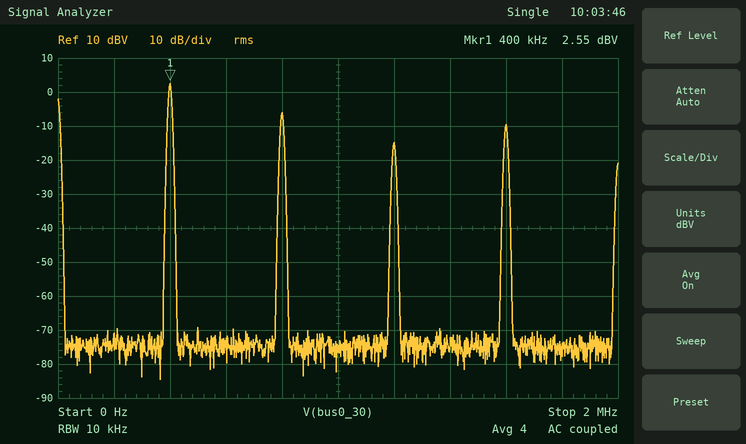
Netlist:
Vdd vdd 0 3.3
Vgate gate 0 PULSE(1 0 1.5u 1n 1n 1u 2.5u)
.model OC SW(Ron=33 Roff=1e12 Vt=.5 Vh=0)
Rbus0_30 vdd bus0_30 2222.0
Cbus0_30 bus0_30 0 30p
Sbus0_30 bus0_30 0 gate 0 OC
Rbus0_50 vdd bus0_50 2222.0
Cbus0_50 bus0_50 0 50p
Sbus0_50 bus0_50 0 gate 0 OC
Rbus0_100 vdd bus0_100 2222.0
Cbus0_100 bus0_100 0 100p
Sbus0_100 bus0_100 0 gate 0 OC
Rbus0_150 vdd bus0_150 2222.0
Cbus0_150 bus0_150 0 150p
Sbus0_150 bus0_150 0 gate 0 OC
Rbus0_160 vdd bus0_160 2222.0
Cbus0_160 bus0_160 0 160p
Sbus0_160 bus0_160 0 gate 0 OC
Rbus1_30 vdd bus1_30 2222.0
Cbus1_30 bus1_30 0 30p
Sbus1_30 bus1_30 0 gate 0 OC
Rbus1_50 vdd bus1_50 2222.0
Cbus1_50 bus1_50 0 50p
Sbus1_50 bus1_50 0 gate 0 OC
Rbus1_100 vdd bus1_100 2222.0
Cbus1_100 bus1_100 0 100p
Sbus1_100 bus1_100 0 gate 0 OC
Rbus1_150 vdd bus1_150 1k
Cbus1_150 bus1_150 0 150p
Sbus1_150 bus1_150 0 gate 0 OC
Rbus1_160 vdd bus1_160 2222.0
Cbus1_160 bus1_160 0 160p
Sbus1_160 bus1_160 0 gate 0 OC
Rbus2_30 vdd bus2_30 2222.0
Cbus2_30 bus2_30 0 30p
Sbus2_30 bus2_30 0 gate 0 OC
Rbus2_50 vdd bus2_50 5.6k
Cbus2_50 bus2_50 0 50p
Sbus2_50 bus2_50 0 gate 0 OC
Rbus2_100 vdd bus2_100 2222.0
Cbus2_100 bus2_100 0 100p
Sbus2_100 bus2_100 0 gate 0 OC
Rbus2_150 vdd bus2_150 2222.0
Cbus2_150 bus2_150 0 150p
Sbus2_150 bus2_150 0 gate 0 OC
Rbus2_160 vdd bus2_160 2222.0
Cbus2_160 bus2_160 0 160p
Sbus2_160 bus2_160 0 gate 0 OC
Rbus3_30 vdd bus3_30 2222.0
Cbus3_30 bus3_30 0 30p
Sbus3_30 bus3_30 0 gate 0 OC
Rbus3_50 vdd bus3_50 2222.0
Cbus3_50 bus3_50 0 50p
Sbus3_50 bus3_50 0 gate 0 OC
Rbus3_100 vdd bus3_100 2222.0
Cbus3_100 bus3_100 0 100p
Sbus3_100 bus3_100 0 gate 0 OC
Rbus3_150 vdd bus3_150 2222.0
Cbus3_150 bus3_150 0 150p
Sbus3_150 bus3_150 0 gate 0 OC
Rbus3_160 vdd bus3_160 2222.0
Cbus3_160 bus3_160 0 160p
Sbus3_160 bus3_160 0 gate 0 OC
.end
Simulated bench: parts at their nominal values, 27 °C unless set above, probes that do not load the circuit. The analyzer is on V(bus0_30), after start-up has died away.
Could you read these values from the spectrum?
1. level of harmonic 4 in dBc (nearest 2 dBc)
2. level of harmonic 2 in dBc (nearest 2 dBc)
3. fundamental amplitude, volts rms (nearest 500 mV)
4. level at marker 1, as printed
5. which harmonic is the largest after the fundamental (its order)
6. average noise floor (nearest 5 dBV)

-12 dBc
-8 dBc
1.5 V
2.55 dBV
2
-75 dBV
